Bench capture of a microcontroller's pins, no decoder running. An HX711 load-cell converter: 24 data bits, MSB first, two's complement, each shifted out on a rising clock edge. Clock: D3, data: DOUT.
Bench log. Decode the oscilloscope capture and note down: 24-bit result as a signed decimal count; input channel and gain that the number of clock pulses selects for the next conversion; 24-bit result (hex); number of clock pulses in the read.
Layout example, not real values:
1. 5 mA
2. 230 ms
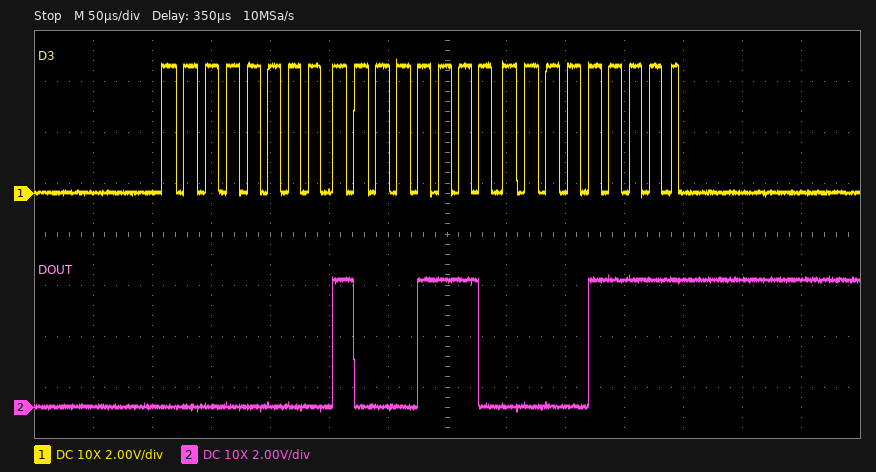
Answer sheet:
1. 36367
2. channel A, gain 128
3. 0x008E0F
4. 25
